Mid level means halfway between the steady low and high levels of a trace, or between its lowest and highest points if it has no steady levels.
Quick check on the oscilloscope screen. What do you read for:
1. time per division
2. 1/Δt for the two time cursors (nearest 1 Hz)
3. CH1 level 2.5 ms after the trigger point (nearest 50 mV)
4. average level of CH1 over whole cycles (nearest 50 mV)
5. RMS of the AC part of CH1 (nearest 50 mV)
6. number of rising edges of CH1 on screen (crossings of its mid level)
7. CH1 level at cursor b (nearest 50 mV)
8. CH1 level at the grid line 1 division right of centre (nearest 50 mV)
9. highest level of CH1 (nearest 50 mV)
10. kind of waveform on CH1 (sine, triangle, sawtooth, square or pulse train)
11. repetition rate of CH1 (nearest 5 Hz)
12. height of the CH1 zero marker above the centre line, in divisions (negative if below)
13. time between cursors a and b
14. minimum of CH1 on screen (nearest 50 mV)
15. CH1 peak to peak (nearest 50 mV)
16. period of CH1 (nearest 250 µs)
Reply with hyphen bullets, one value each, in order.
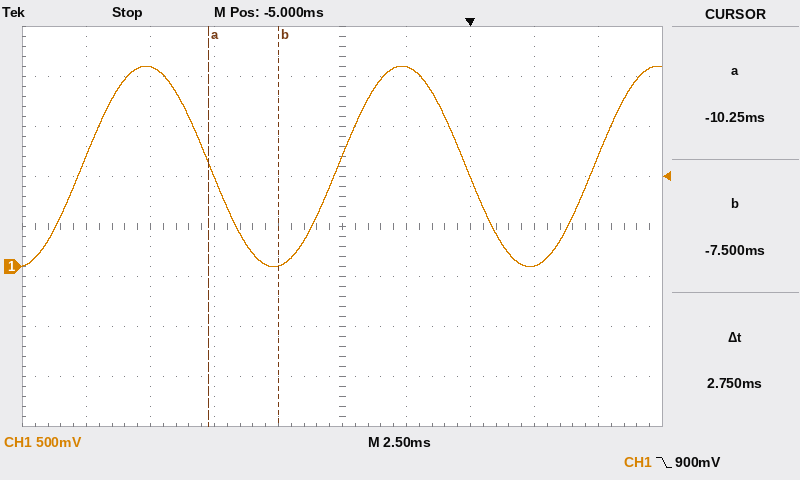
- 2.5 ms
- 364 Hz
- 0 mV
- 1.00 V
- 700 mV
- 3
- 0 mV
- 2.00 V
- 2.00 V
- sine
- 100 Hz
- -0.8 div
- 2.75 ms
- 0 mV
- 2.00 V
- 10.00 ms
